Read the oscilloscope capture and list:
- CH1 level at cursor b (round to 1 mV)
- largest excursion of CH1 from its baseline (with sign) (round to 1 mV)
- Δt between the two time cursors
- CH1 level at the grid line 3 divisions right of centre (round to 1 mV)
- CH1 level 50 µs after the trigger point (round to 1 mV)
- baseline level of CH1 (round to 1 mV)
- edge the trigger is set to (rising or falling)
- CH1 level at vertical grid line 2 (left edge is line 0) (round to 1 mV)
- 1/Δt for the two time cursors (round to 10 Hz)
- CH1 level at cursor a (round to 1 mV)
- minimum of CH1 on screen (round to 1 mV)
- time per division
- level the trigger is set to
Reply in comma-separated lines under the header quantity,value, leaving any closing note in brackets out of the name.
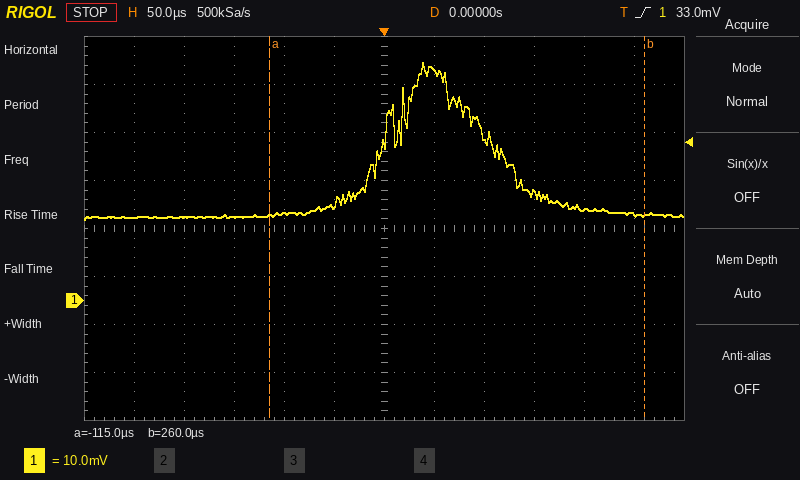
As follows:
quantity,value
CH1 level at cursor b,18 mV
largest excursion of CH1 from its baseline (with sign),+32 mV
Δt between the two time cursors,375 µs
CH1 level at the grid line 3 divisions right of centre,22 mV
CH1 level 50 µs after the trigger point,48 mV
baseline level of CH1,18 mV
edge the trigger is set to,rising
CH1 level at vertical grid line 2 (left edge is line 0),17 mV
1/Δt for the two time cursors,2.67 kHz
CH1 level at cursor a,18 mV
minimum of CH1 on screen,17 mV
time per division,50 µs
level the trigger is set to,33.0 mV
